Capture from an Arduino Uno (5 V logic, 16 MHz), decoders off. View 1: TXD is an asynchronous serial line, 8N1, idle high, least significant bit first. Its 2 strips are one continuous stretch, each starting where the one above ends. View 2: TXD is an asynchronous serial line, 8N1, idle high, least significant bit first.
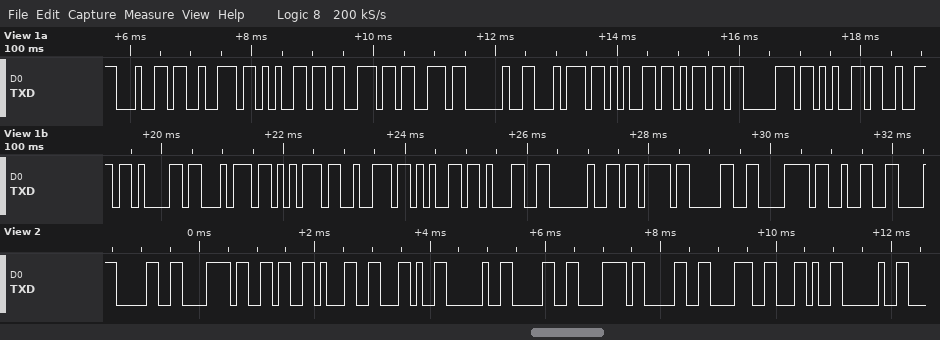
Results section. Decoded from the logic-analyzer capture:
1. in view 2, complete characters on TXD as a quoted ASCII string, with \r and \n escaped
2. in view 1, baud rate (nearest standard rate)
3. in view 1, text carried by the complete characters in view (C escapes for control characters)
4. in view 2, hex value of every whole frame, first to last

"0x61, 0x08, "
9600 baud
"dress temperature1 {0x2"
30 78 36 31 2C 20 30 78 30 38 2C 20
